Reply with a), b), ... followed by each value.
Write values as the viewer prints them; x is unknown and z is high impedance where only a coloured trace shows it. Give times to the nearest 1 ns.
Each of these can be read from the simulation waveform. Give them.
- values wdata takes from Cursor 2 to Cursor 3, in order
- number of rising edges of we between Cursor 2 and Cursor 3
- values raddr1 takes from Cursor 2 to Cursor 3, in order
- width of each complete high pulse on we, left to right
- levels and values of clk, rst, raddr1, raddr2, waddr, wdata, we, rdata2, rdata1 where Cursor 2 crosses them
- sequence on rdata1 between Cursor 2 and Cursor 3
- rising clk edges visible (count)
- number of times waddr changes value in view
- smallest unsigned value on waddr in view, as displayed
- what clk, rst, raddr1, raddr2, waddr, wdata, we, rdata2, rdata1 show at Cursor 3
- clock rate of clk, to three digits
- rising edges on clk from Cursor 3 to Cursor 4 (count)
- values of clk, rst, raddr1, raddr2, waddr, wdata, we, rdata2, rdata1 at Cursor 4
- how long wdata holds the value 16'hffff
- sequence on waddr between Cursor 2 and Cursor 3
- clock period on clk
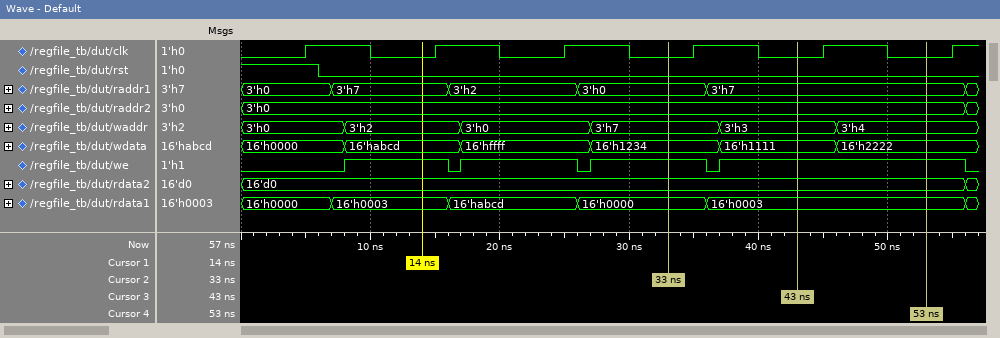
a) 16'h1234, 16'h1111
b) 1
c) 3'h0, 3'h7
d) 8 ns, 9 ns, 9 ns, 19 ns
e) clk=0, rst=0, raddr1=3'h0, raddr2=3'h0, waddr=3'h7, wdata=16'h1234, we=1, rdata2=16'd0, rdata1=16'h0000
f) 16'h0000, 16'h0003
g) 6
h) 5
i) 3'h0
j) clk=0, rst=0, raddr1=3'h7, raddr2=3'h0, waddr=3'h3, wdata=16'h1111, we=1, rdata2=16'd0, rdata1=16'h0003
k) 100 MHz
l) 1
m) clk=0, rst=0, raddr1=3'h7, raddr2=3'h0, waddr=3'h4, wdata=16'h2222, we=1, rdata2=16'd0, rdata1=16'h0003
n) 10 ns
o) 3'h7, 3'h3
p) 10 ns
